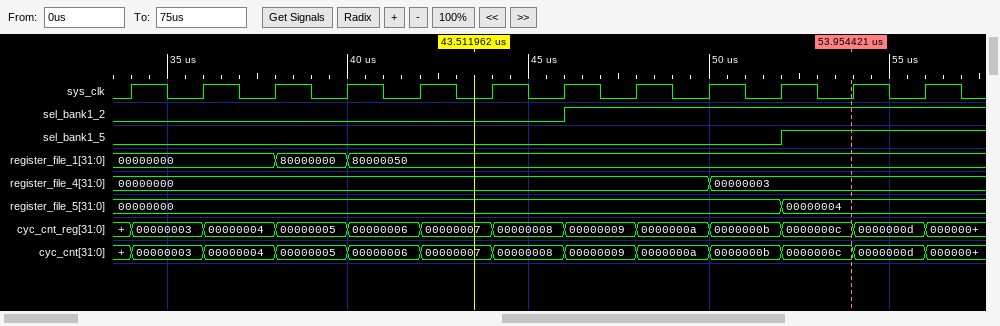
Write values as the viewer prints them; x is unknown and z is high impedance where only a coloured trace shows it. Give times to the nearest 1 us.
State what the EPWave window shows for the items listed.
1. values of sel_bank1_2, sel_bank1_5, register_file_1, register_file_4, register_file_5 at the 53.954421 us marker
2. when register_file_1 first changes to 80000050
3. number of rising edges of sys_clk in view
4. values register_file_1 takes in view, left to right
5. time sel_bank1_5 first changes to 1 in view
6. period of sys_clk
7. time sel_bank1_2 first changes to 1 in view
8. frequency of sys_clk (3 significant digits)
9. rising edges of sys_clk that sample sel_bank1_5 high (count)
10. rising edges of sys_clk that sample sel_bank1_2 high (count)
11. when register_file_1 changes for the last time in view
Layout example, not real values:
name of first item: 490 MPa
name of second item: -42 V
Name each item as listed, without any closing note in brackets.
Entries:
values of sel_bank1_2, sel_bank1_5, register_file_1, register_file_4, register_file_5 at the 53.954421 us marker: sel_bank1_2=1, sel_bank1_5=1, register_file_1=80000050, register_file_4=00000003, register_file_5=00000004
when register_file_1 first changes to 80000050: 40 us
number of rising edges of sys_clk in view: 12
values register_file_1 takes in view, left to right: 00000000, 80000000, 80000050
time sel_bank1_5 first changes to 1 in view: 52 us
period of sys_clk: 2 us
time sel_bank1_2 first changes to 1 in view: 46 us
frequency of sys_clk: 500 kHz
rising edges of sys_clk that sample sel_bank1_5 high: 2
rising edges of sys_clk that sample sel_bank1_2 high: 5
when register_file_1 changes for the last time in view: 40 us
